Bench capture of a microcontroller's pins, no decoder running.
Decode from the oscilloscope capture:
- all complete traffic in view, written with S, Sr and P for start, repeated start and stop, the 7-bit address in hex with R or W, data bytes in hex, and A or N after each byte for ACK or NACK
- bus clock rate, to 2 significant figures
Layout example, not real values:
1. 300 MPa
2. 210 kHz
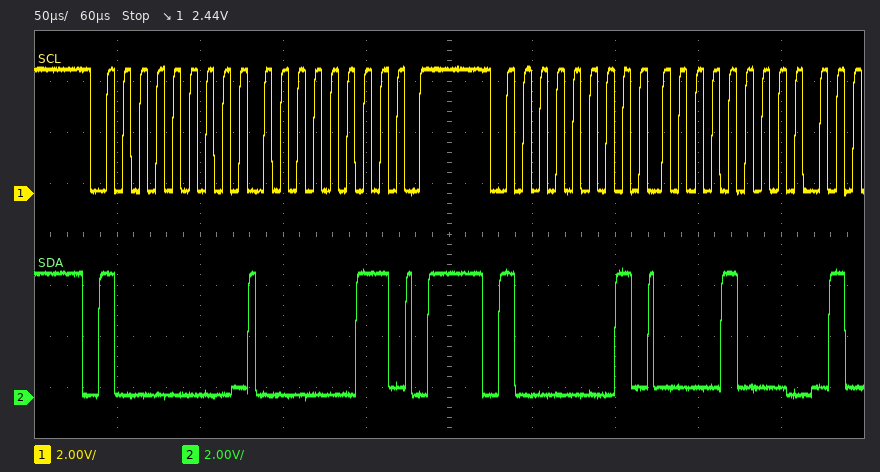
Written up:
1. S 40W A 03 A P S 40R A 08 A
2. 100 kHz
